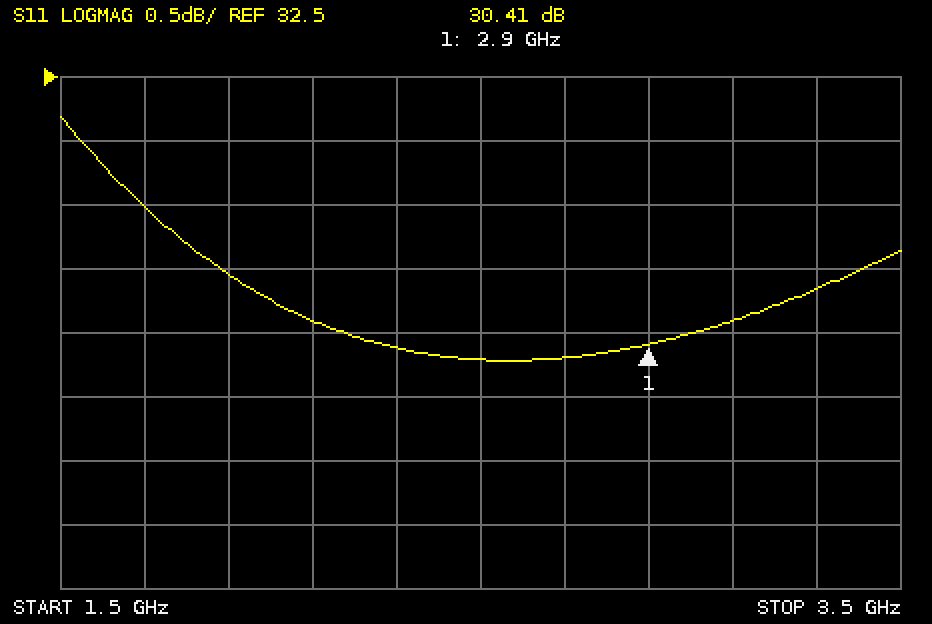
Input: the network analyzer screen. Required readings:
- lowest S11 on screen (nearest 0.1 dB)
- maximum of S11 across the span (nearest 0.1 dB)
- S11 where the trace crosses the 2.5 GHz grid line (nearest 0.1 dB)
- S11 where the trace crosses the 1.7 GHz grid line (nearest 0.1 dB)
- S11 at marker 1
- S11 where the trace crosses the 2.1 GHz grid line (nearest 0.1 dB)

30.3 dB
32.2 dB
30.3 dB
31.5 dB
30.41 dB
30.6 dB
